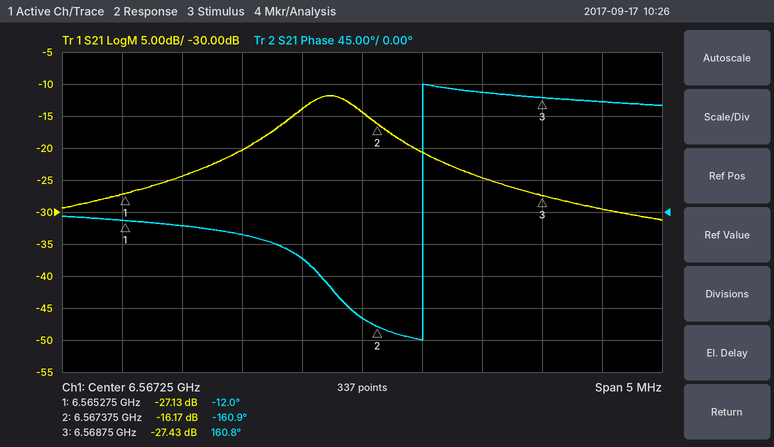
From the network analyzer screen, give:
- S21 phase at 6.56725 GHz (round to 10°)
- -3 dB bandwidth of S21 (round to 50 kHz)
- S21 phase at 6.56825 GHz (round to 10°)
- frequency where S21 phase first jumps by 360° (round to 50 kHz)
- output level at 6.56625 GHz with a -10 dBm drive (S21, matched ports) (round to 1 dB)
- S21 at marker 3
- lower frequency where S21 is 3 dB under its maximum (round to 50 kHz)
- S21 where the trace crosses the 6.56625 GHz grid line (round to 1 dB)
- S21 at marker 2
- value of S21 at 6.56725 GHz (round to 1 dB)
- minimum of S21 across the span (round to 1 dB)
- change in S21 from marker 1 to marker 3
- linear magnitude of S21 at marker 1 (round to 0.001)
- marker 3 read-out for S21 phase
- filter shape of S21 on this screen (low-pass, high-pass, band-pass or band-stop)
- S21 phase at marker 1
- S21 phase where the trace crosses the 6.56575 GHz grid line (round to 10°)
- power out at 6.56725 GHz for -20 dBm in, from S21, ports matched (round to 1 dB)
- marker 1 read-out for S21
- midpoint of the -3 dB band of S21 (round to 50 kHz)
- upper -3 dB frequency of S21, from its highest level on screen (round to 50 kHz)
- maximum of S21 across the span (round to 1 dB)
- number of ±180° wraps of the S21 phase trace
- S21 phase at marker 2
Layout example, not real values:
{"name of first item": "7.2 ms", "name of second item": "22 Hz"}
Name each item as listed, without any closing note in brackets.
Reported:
{"S21 phase at 6.56725 GHz": "-150°", "-3 dB bandwidth of S21": "600 kHz", "S21 phase at 6.56825 GHz": "170°", "frequency where S21 phase first jumps by 360°": "6.56775 GHz", "output level at 6.56625 GHz with a -10 dBm drive (S21, matched ports)": "-30 dBm", "S21 at marker 3": "-27.43 dB", "lower frequency where S21 is 3 dB under its maximum": "6.56670 GHz", "S21 where the trace crosses the 6.56625 GHz grid line": "-20 dB", "S21 at marker 2": "-16.17 dB", "value of S21 at 6.56725 GHz": "-14 dB", "minimum of S21 across the span": "-31 dB", "change in S21 from marker 1 to marker 3": "-0.30 dB", "linear magnitude of S21 at marker 1": "0.044", "marker 3 read-out for S21 phase": "160.8°", "filter shape of S21 on this screen": "band-pass", "S21 phase at marker 1": "-12.0°", "S21 phase where the trace crosses the 6.56575 GHz grid line": "-20°", "power out at 6.56725 GHz for -20 dBm in, from S21, ports matched": "-34 dBm", "marker 1 read-out for S21": "-27.13 dB", "midpoint of the -3 dB band of S21": "6.56700 GHz", "upper -3 dB frequency of S21, from its highest level on screen": "6.56730 GHz", "maximum of S21 across the span": "-12 dB", "number of ±180° wraps of the S21 phase trace": "1", "S21 phase at marker 2": "-160.9°"}
